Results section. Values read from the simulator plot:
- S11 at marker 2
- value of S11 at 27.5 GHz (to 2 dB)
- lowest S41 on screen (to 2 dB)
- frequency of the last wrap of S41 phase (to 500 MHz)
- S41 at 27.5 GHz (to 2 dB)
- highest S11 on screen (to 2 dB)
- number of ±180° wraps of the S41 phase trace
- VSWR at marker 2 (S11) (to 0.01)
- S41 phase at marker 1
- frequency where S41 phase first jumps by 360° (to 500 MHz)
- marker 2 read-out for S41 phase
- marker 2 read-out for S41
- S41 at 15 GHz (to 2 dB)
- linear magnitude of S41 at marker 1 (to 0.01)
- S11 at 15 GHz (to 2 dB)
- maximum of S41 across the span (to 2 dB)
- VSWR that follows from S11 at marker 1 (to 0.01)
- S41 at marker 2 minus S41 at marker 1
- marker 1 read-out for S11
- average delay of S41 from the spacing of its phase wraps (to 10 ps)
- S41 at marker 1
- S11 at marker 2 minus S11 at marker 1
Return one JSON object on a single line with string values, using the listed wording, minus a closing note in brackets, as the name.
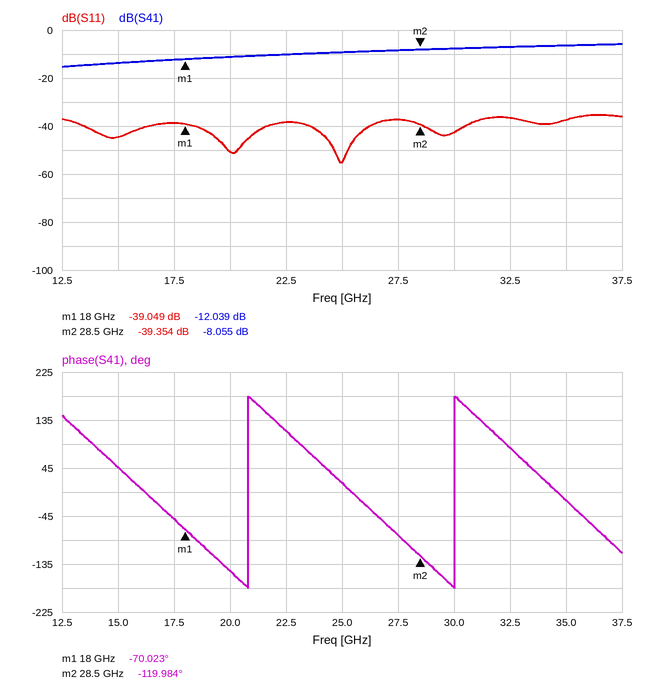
{"S11 at marker 2": "-39.354 dB", "value of S11 at 27.5 GHz": "-38 dB", "lowest S41 on screen": "-16 dB", "frequency of the last wrap of S41 phase": "30.0 GHz", "S41 at 27.5 GHz": "-8 dB", "highest S11 on screen": "-36 dB", "number of ±180° wraps of the S41 phase trace": "2", "VSWR at marker 2 (S11)": "1.02", "S41 phase at marker 1": "-70.023°", "frequency where S41 phase first jumps by 360°": "21.0 GHz", "marker 2 read-out for S41 phase": "-119.984°", "marker 2 read-out for S41": "-8.055 dB", "S41 at 15 GHz": "-14 dB", "linear magnitude of S41 at marker 1": "0.25", "S11 at 15 GHz": "-44 dB", "maximum of S41 across the span": "-6 dB", "VSWR that follows from S11 at marker 1": "1.02", "S41 at marker 2 minus S41 at marker 1": "3.984 dB", "marker 1 read-out for S11": "-39.049 dB", "average delay of S41 from the spacing of its phase wraps": "110 ps", "S41 at marker 1": "-12.039 dB", "S11 at marker 2 minus S11 at marker 1": "-0.305 dB"}
